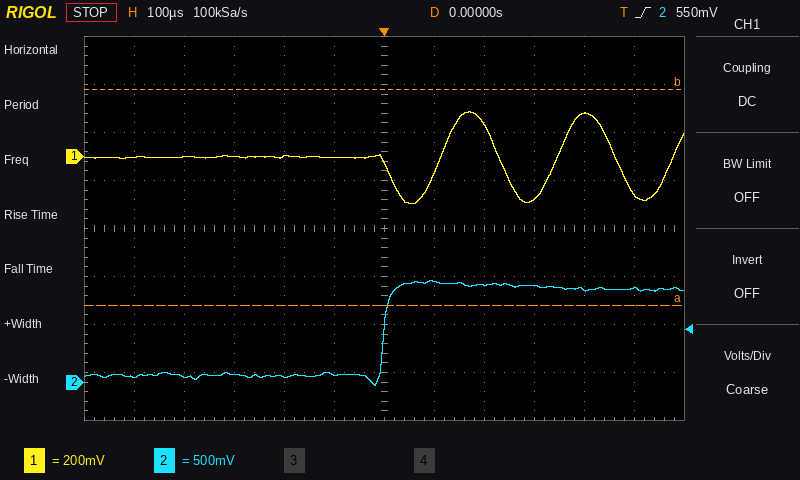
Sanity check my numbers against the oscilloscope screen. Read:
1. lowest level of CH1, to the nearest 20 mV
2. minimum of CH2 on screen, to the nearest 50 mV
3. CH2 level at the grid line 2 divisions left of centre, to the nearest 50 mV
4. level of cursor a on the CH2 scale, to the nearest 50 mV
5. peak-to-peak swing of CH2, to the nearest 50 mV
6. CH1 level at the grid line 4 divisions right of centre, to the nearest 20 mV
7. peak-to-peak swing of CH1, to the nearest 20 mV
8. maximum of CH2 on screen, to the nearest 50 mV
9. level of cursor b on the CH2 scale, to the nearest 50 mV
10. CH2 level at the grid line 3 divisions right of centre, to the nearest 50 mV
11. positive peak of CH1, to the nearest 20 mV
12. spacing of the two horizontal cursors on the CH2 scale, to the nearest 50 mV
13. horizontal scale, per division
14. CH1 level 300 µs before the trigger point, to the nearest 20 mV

-200 mV
-50 mV
50 mV
800 mV
1.10 V
180 mV
380 mV
1.05 V
3.05 V
1.00 V
180 mV
2.25 V
100 µs
0 mV
